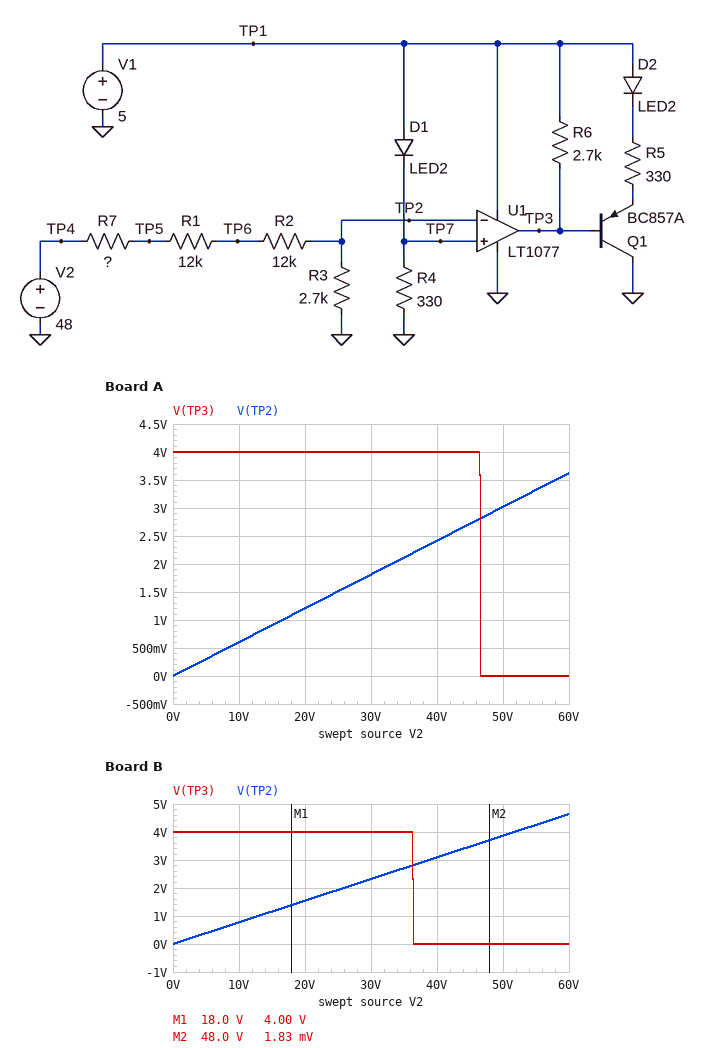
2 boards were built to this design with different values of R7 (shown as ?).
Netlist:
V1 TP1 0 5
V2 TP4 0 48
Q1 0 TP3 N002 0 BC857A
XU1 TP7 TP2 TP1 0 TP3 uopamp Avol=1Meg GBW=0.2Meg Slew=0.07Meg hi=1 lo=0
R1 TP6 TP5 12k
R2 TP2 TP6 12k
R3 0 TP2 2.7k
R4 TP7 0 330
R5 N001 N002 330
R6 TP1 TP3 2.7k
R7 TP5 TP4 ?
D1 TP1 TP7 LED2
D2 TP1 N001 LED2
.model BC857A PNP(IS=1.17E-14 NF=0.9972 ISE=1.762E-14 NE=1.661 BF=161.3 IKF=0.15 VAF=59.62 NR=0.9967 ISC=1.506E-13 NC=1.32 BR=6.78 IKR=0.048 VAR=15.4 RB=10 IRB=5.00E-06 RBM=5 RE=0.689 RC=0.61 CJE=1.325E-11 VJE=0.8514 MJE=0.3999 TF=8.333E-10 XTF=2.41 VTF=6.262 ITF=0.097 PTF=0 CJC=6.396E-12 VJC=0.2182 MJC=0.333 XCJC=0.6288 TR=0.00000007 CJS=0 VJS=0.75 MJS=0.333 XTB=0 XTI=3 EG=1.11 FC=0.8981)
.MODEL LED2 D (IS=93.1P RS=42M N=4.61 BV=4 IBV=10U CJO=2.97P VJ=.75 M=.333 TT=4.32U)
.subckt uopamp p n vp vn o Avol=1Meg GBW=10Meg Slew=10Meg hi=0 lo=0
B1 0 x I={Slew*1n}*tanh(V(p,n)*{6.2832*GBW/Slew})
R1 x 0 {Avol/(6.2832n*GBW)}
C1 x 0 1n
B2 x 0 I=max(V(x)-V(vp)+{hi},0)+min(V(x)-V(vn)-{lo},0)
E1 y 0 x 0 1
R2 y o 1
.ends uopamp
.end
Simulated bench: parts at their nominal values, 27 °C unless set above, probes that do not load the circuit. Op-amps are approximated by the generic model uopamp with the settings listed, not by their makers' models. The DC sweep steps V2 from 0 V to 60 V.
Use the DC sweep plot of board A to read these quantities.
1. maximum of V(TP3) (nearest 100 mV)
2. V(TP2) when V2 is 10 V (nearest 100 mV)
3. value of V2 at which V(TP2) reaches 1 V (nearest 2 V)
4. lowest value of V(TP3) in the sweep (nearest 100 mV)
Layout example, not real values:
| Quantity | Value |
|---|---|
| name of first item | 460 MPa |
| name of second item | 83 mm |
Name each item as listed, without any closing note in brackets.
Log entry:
| Quantity | Value |
|---|---|
| maximum of V(TP3) | 4.0 V |
| V(TP2) when V2 is 10 V | 600 mV |
| value of V2 at which V(TP2) reaches 1 V | 16 V |
| lowest value of V(TP3) in the sweep | 0 V |
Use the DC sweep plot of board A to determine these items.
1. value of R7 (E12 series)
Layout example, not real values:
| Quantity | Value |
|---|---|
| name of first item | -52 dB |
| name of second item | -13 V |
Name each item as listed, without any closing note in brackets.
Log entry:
| Quantity | Value |
|---|---|
| value of R7 | 18 kΩ |
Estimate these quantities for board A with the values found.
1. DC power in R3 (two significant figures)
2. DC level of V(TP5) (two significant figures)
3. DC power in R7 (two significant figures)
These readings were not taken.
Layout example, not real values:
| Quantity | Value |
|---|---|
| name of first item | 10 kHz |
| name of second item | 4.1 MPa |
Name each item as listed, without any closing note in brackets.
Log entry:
| Quantity | Value |
|---|---|
| DC power in R3 | 3.1 mW |
| DC level of V(TP5) | 29 V |
| DC power in R7 | 21 mW |
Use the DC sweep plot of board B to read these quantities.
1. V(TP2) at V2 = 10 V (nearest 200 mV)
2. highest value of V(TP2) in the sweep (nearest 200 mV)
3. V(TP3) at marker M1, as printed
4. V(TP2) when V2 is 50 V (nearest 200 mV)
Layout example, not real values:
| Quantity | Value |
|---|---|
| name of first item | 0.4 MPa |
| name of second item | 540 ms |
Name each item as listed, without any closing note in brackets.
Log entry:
| Quantity | Value |
|---|---|
| V(TP2) at V2 = 10 V | 800 mV |
| highest value of V(TP2) in the sweep | 4.6 V |
| V(TP3) at marker M1, as printed | 4.00 V |
| V(TP2) when V2 is 50 V | 3.8 V |
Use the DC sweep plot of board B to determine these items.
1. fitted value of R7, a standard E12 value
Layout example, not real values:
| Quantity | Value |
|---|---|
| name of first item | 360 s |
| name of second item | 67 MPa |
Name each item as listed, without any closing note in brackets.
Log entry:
| Quantity | Value |
|---|---|
| fitted value of R7, a standard E12 value | 8.2 kΩ |
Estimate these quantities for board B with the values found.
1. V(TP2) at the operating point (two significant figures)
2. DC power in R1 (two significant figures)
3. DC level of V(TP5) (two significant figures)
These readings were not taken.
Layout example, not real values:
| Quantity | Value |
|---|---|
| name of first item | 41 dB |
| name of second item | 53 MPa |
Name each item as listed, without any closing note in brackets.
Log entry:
| Quantity | Value |
|---|---|
| V(TP2) at the operating point | 3.7 V |
| DC power in R1 | 23 mW |
| DC level of V(TP5) | 37 V |
